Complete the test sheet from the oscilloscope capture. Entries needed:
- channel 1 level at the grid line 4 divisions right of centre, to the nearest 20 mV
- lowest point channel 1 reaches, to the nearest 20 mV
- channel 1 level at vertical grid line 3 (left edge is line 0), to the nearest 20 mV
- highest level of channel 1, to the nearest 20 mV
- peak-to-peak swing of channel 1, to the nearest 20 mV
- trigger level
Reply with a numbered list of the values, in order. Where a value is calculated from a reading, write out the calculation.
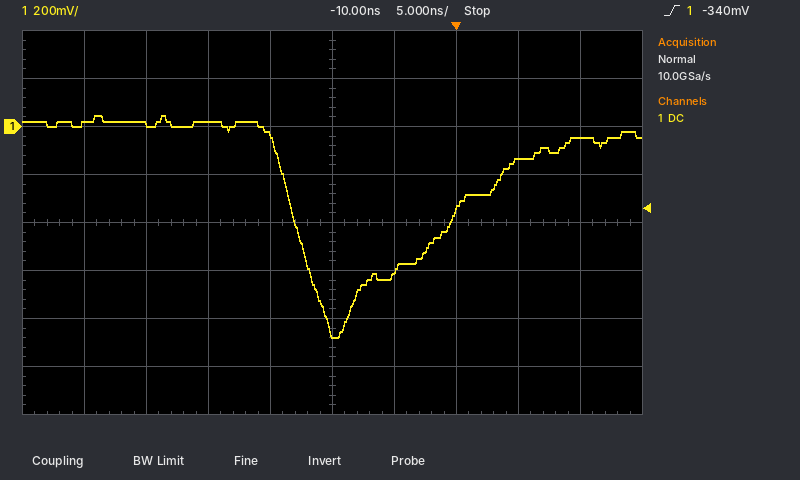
1. -40 mV
2. -880 mV
3. 20 mV
4. 40 mV
5. 40 mV − (-880 mV) = 920 mV
6. -340 mV
